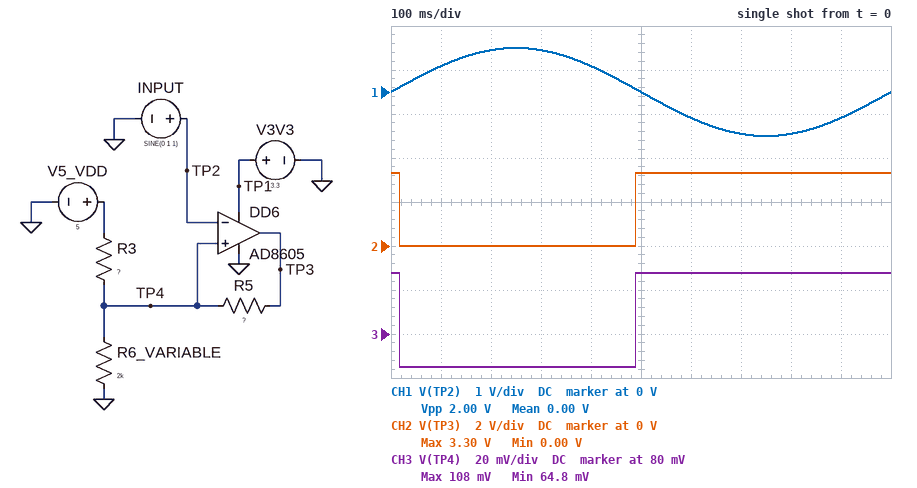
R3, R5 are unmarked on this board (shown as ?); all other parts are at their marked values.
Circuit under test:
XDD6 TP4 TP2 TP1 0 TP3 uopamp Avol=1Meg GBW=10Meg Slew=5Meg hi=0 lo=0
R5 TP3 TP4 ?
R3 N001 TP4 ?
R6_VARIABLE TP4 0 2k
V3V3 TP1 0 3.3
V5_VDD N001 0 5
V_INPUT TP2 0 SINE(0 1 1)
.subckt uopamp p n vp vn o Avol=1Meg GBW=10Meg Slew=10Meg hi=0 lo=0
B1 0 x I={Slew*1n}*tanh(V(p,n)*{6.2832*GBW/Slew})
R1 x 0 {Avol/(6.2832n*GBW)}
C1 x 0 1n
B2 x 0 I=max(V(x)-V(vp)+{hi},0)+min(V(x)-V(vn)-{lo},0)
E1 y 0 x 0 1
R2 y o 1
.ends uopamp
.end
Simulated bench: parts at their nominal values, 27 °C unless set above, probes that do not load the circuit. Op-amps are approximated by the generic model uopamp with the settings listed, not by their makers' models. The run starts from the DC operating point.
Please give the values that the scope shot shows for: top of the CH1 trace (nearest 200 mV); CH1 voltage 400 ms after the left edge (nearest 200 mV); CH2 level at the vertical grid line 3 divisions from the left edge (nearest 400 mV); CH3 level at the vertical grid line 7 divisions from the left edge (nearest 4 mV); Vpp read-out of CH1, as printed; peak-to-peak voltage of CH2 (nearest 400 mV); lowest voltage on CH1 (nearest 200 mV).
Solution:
1.0 V
600 mV
0 V
108 mV
2.00 V
3.2 V
-1.0 V
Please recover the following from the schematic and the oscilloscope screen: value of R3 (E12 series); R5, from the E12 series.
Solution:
150 kΩ
150 kΩ
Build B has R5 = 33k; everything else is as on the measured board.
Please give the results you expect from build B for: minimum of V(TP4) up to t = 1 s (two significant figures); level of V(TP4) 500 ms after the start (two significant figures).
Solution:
62 mV
250 mV
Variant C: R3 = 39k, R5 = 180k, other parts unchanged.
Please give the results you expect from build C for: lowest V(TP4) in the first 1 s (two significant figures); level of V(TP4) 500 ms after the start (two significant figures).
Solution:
240 mV
280 mV
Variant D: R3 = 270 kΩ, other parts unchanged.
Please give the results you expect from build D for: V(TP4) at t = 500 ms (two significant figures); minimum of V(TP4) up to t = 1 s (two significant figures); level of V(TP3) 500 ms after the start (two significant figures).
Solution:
79 mV
36 mV
3.3 V
